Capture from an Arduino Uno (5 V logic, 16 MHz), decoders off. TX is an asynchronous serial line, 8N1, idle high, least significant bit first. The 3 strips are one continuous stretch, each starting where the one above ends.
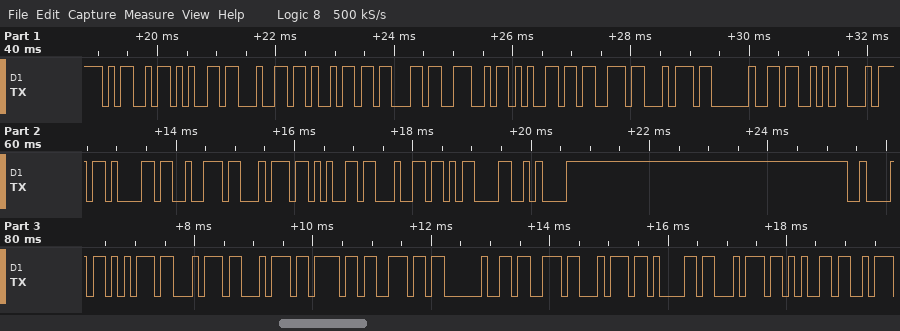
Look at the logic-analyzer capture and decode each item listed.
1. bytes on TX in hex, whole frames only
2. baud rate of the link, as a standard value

4D 65 64 69 63 4E 65 73 74 20 53 74 61 72 74 65 64 0D 0A 42 75 74 74 6F 6E 20 73 74 61 74 65
9600 baud
